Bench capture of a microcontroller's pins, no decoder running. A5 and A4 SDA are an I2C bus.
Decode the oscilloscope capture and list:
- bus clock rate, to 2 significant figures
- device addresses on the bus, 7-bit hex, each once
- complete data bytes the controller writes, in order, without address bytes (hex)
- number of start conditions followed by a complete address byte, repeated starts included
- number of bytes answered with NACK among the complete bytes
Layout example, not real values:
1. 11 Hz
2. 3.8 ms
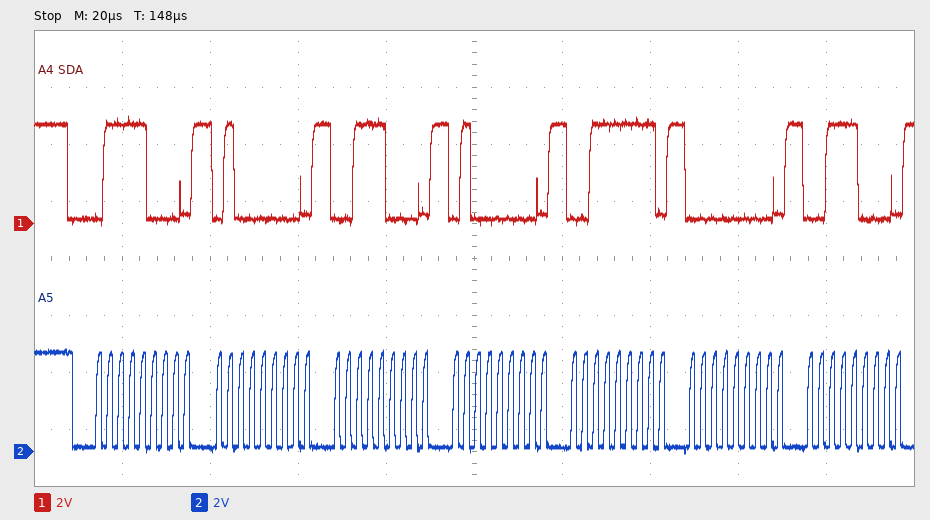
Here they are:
1. 400 kHz
2. 0x3C
3. 40 38 40 3F 00 38
4. 1
5. 0
